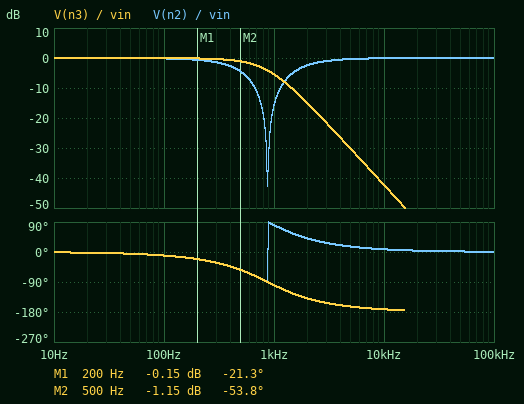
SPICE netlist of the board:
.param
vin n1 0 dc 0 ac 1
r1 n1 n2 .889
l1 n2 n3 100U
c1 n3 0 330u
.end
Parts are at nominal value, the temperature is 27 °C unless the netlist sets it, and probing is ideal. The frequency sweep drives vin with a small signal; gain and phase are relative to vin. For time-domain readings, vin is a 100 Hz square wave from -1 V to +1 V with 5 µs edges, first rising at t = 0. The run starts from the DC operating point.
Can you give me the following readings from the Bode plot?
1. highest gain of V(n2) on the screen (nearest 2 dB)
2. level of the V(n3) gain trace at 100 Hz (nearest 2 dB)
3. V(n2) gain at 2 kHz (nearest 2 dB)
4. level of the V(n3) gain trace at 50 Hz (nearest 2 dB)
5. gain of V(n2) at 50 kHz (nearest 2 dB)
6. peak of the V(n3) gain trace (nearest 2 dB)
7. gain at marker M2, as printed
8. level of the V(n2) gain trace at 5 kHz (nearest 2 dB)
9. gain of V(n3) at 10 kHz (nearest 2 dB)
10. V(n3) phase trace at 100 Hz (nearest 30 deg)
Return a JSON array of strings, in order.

["0 dB", "0 dB", "-2 dB", "0 dB", "0 dB", "0 dB", "-1.15 dB", "0 dB", "-42 dB", "0 deg"]
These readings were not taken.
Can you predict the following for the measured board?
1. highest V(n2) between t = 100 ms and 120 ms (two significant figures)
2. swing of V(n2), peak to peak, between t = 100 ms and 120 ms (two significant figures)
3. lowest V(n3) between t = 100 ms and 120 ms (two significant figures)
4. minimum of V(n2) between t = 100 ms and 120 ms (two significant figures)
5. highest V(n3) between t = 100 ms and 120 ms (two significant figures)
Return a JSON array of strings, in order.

["1.0 V", "2.0 V", "-1.0 V", "-1.0 V", "1.0 V"]
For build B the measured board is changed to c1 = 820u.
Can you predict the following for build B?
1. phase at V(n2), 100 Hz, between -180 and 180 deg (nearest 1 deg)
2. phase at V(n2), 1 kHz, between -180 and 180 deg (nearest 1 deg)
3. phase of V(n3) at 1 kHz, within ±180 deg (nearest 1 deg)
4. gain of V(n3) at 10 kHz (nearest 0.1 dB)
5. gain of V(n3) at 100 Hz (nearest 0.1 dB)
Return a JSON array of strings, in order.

["-25 deg", "64 deg", "-116 deg", "-50.3 dB", "-0.6 dB"]
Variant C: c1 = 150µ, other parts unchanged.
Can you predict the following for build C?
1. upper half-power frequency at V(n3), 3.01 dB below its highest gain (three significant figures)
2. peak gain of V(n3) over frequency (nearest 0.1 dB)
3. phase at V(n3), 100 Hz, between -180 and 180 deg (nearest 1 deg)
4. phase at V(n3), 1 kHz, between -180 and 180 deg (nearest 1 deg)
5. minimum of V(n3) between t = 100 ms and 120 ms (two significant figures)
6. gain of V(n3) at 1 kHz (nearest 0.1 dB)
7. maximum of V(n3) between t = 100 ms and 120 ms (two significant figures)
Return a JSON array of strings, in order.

["1.49 kHz", "0.8 dB", "-5 deg", "-64 deg", "-1.3 V", "0.6 dB", "1.3 V"]
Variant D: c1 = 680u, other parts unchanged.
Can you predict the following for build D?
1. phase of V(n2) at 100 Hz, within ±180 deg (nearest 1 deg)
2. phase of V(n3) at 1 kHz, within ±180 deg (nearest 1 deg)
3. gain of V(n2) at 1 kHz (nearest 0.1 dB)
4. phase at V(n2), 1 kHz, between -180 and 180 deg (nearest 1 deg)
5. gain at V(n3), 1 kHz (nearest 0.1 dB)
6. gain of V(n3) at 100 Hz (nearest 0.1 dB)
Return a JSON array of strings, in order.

["-21 deg", "-114 deg", "-7.8 dB", "66 deg", "-12.4 dB", "-0.4 dB"]
